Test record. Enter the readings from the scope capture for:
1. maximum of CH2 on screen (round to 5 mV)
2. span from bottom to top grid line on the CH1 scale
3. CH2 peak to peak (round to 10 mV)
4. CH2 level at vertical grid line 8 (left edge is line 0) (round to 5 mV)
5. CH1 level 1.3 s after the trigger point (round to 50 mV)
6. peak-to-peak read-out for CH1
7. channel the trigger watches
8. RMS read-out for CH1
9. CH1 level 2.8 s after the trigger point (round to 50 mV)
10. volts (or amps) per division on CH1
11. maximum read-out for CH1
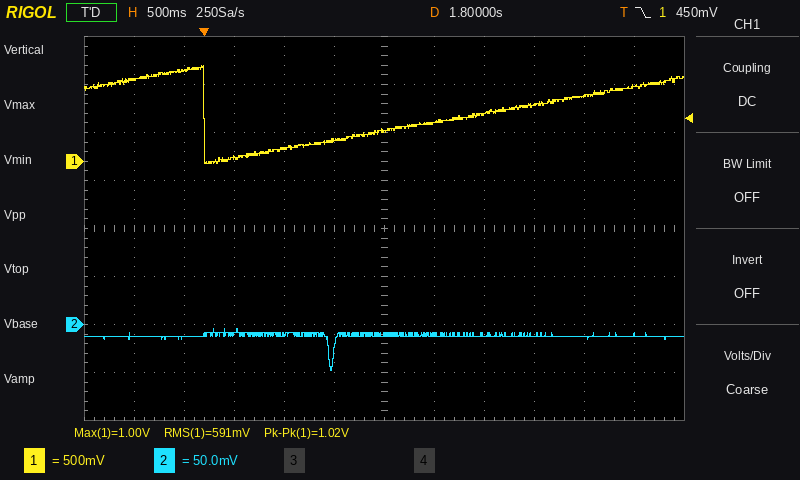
-5 mV
4 V
40 mV
-10 mV
200 mV
1.02 V
CH1
591 mV
500 mV
500 mV
1.00 V
